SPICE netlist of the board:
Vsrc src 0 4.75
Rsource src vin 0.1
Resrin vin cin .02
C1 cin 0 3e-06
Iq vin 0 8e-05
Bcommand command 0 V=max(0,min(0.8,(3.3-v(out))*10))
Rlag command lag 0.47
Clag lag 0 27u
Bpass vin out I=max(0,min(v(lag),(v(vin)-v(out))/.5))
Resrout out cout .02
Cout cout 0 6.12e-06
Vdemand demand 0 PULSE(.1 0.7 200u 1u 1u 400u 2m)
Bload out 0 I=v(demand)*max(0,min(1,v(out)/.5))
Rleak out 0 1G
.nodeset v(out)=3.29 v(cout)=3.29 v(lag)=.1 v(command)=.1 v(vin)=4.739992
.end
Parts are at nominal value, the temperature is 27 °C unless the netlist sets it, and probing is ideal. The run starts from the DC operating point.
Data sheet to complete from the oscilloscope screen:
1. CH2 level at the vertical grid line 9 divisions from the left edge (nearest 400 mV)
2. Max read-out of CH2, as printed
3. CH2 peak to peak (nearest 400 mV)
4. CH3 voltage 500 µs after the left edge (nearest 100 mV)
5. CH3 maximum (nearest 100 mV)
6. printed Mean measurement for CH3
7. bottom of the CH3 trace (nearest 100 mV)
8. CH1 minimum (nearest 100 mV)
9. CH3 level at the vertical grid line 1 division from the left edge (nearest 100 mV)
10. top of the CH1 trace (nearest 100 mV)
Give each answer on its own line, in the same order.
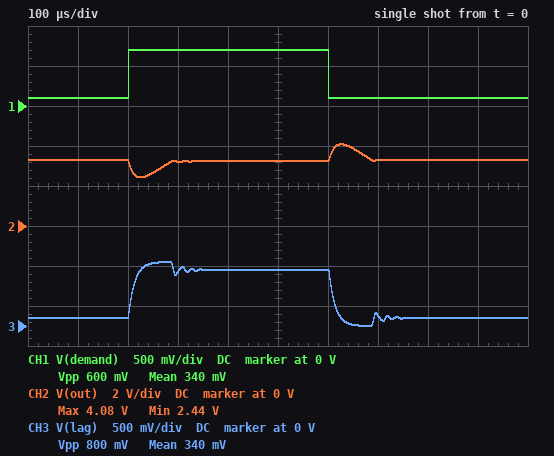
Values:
3.2 V
4.08 V
1.6 V
700 mV
800 mV
340 mV
0 V
100 mV
100 mV
700 mV
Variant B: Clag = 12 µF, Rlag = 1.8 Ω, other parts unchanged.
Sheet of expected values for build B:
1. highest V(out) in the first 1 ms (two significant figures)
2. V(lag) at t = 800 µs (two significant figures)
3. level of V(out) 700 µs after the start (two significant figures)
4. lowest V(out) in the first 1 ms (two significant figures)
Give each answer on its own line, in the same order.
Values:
4.7 V
130 mV
4.1 V
1.8 V
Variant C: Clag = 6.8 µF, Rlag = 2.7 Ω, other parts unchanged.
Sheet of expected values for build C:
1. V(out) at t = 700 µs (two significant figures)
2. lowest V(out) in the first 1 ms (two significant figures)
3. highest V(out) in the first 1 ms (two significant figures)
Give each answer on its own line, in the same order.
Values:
3.7 V
2.1 V
4.5 V
